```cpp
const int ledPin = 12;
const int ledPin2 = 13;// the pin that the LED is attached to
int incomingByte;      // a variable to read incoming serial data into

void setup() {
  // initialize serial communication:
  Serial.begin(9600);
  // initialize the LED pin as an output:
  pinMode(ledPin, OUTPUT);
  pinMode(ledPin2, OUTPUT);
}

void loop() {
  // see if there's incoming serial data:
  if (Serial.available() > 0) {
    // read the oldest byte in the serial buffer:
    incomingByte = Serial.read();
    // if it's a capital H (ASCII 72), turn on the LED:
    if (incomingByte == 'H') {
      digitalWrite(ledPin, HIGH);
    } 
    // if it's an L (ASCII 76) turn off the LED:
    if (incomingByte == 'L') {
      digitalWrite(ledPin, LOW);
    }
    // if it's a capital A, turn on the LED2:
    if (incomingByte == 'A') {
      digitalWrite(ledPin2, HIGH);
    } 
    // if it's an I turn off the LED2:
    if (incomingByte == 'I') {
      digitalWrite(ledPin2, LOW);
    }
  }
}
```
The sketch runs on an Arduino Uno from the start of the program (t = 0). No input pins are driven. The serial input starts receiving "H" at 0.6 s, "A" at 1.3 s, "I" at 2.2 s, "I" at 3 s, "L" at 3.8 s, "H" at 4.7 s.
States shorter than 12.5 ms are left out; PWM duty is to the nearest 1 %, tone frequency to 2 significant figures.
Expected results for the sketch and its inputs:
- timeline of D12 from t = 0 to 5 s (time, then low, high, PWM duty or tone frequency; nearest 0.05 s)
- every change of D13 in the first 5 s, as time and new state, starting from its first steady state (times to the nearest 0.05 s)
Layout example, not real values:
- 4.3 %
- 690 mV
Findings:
- 0 s low; 0.6 s high; 3.8 s low; 4.7 s high
- 0 s low; 1.3 s high; 2.2 s low
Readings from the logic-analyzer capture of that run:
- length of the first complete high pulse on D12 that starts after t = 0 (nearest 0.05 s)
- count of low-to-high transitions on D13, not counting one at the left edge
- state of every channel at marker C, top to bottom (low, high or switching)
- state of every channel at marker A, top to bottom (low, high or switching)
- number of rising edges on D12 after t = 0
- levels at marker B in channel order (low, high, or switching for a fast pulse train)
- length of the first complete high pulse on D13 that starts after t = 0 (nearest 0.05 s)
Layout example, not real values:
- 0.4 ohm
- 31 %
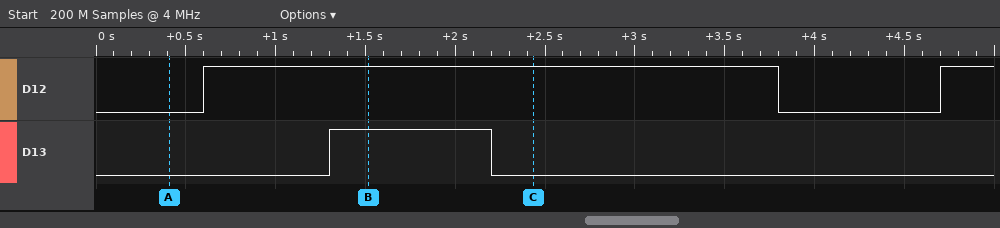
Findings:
- 3.20 s
- 1
- D12 high, D13 low
- D12 low, D13 low
- 2
- D12 high, D13 high
- 0.90 s
